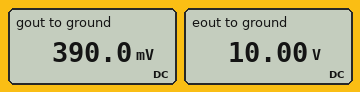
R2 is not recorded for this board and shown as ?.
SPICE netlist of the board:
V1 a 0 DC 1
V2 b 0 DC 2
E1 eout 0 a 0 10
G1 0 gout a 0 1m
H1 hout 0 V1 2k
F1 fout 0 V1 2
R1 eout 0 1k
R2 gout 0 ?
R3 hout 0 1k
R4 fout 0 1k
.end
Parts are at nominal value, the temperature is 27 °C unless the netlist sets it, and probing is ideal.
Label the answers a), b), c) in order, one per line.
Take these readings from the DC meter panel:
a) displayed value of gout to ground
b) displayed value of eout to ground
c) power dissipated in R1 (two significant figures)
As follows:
a) 390.0 mV
b) 10.00 V
c) 100 mW
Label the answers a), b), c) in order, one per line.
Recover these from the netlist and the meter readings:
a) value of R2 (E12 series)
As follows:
a) 390 Ω
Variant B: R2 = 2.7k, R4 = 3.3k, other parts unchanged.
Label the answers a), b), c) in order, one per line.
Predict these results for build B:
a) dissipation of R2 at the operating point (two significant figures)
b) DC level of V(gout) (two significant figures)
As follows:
a) 2.7 mW
b) 2.7 V
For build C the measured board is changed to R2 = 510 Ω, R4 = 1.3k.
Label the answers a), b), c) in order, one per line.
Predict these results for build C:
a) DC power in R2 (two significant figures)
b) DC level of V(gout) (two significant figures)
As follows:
a) 510 µW
b) 510 mV
